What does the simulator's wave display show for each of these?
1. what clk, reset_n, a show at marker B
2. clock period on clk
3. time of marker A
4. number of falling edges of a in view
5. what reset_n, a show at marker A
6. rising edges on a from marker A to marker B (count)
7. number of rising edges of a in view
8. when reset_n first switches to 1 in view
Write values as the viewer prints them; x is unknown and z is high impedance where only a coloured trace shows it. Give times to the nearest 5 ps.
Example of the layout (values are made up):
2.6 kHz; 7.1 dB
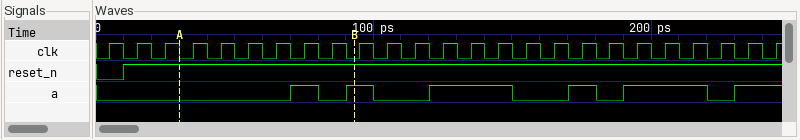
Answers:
clk=0, reset_n=1, a=1; 10 ps; 30 ps; 5; reset_n=1, a=0; 2; 6; 10 ps
